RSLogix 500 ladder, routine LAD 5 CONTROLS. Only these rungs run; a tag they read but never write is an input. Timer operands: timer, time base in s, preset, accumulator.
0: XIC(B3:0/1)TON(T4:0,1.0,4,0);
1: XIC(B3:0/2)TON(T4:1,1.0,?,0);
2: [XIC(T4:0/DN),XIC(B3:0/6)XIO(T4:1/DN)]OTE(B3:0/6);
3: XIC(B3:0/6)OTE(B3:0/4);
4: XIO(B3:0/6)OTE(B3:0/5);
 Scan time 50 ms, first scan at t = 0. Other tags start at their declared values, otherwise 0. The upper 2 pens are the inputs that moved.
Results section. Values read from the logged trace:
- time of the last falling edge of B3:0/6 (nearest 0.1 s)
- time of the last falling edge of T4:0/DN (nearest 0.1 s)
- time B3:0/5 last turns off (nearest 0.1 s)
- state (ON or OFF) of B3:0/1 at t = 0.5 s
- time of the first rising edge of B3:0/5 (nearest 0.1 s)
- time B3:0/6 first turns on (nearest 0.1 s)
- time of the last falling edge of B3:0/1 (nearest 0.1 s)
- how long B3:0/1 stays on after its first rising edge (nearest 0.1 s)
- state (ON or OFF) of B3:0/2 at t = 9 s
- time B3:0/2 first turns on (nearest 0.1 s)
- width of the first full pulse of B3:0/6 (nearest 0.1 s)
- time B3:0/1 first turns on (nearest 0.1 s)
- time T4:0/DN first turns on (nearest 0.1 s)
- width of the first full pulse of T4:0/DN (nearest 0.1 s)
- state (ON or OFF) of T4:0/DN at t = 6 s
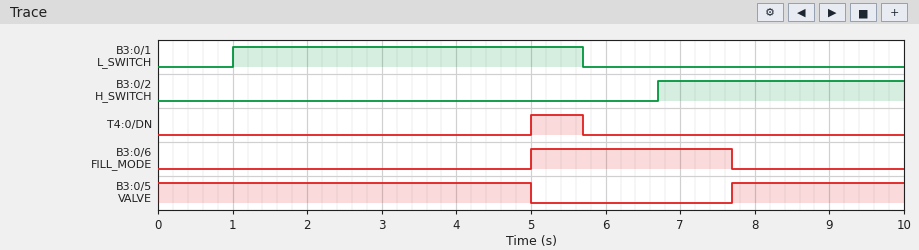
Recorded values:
7.7 s
5.7 s
5.0 s
OFF
7.7 s
5.0 s
5.7 s
4.7 s
ON
6.7 s
2.7 s
1.0 s
5.0 s
0.7 s
OFF
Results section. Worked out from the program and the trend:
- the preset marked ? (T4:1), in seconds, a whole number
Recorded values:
1 s
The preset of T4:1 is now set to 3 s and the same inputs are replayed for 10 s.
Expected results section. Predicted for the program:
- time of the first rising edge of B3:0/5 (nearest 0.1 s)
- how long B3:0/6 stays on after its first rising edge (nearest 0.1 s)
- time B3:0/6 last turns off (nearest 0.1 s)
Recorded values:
9.7 s
4.7 s
9.7 s
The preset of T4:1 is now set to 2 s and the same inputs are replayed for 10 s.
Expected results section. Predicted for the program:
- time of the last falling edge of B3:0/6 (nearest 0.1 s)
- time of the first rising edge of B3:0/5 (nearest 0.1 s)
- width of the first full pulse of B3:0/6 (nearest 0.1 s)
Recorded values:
8.7 s
8.7 s
3.7 s
